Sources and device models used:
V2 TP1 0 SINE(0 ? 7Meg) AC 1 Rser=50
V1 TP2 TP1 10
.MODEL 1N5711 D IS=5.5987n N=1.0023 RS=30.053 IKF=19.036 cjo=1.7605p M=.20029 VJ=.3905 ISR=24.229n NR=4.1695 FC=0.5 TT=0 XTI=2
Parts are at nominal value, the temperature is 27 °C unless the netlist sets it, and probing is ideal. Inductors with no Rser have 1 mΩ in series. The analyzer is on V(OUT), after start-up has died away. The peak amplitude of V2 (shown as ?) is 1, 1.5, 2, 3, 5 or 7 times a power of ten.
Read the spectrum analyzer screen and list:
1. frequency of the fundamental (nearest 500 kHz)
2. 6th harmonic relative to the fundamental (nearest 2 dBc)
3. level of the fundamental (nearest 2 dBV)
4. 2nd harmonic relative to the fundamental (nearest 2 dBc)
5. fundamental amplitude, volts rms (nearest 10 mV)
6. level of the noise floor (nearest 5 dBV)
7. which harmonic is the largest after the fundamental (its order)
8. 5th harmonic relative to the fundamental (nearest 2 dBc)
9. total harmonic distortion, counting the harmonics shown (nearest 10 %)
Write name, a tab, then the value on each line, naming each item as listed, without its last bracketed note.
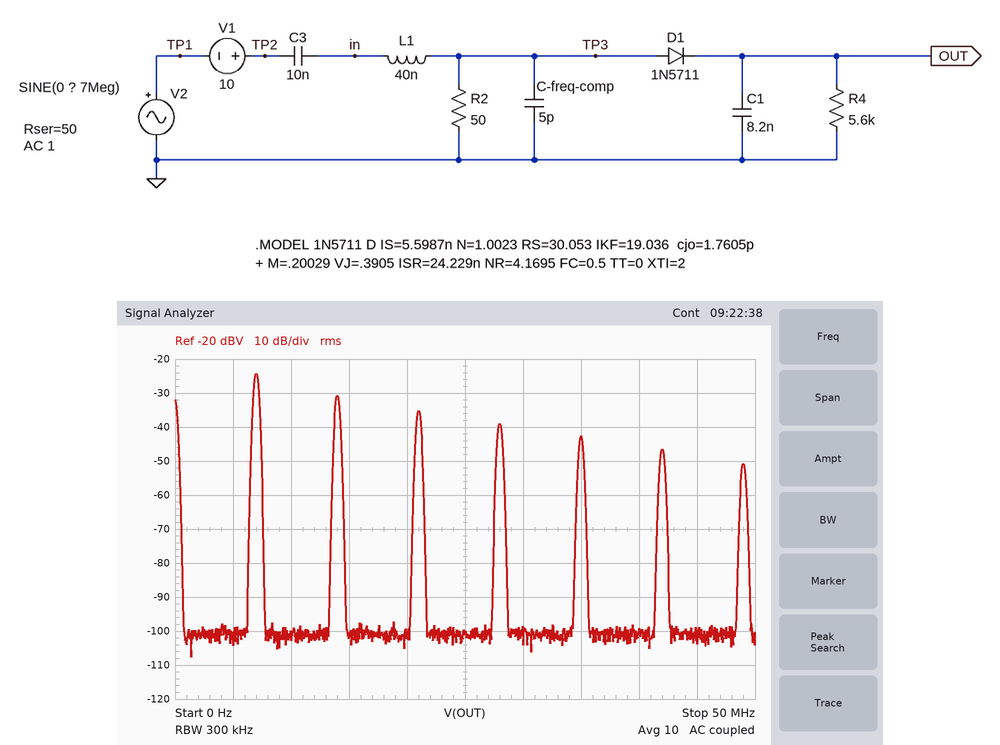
frequency of the fundamental	7.0 MHz
6th harmonic relative to the fundamental	-22 dBc
level of the fundamental	-24 dBV
2nd harmonic relative to the fundamental	-6 dBc
fundamental amplitude, volts rms	60 mV
level of the noise floor	-100 dBV
which harmonic is the largest after the fundamental	2
5th harmonic relative to the fundamental	-18 dBc
total harmonic distortion, counting the harmonics shown	60 %
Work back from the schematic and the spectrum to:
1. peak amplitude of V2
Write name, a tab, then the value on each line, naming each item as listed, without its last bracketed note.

peak amplitude of V2	200 V
